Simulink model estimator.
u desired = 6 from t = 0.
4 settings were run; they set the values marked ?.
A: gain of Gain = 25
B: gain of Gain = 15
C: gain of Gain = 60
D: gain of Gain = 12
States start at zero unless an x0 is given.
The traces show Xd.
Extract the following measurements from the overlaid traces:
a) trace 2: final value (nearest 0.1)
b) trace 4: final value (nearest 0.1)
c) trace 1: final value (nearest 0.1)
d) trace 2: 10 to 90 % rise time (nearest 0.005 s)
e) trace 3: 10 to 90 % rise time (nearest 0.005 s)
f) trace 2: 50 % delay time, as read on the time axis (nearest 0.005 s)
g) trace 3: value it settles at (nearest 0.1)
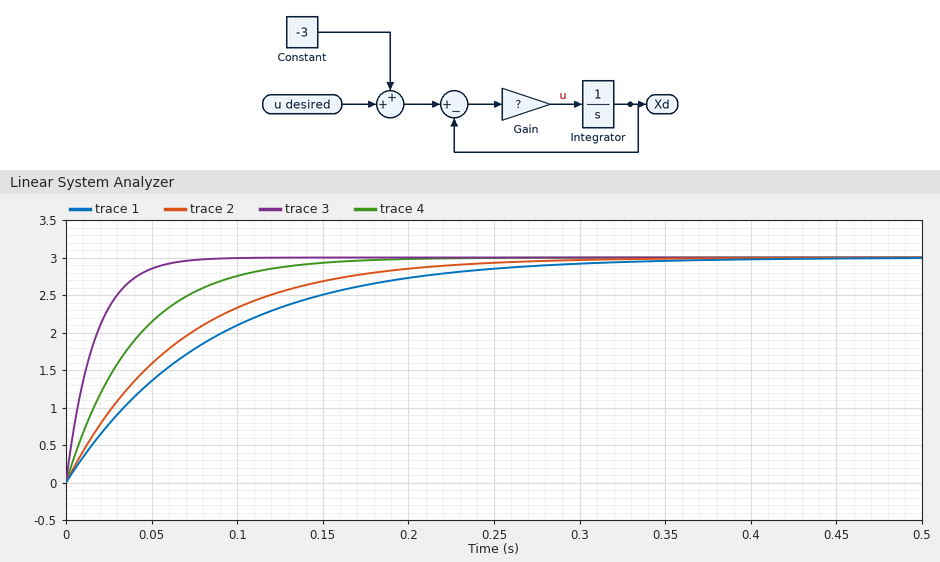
3.0
3.0
3.0
0.145 s
0.035 s
0.045 s
3.0
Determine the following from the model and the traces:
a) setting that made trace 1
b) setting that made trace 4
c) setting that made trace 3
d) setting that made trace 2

D
A
C
B
